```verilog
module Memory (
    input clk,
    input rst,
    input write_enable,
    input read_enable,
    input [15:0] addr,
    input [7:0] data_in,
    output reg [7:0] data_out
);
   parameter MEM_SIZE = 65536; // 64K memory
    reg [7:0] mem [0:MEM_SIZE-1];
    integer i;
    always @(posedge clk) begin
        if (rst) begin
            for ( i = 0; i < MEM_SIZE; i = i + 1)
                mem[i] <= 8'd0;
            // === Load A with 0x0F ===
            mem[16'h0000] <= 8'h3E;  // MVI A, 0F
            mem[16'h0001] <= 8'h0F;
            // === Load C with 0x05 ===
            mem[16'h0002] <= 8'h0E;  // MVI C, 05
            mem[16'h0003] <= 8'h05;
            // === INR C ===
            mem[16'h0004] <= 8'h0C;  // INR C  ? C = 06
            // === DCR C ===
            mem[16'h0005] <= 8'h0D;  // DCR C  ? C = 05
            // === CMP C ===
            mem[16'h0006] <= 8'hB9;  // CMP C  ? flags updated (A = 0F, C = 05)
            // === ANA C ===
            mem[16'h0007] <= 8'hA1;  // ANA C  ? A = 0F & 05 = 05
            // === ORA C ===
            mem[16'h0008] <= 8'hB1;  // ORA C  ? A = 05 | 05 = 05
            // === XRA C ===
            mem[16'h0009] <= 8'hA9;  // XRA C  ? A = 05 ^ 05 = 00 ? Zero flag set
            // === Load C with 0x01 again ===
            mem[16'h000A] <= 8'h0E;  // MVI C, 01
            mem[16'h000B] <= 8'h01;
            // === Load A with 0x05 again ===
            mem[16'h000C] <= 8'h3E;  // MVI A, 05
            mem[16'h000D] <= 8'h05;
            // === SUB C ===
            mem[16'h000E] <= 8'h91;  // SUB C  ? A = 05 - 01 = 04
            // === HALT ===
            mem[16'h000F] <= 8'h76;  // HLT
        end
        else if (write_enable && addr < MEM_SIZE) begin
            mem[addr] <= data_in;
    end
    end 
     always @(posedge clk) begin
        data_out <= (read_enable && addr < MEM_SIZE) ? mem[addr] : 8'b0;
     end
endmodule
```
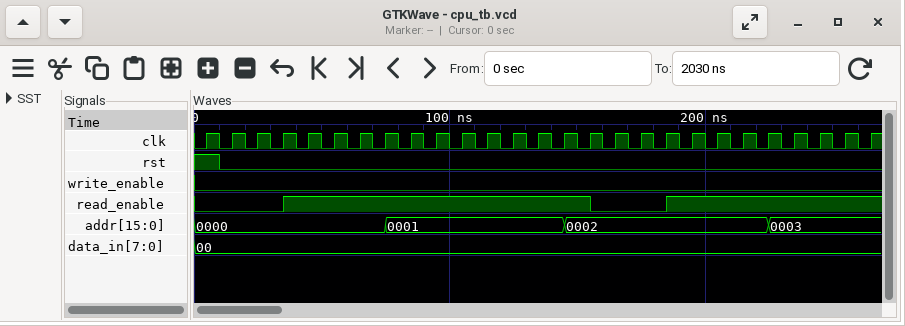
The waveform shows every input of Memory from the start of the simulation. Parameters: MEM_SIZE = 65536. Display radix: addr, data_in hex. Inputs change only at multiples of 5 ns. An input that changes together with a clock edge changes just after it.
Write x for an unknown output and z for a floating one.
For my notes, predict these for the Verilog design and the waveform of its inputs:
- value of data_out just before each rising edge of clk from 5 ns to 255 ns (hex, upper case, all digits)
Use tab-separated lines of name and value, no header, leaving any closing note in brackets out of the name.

value of data_out just before each rising edge of clk from 5 ns to 255 ns	x, 00, 00, 00, 00, 3E, 3E, 3E, 3E, 0F, 0F, 0F, 0F, 0F, 0F, 0F, 0E, 00, 00, 00, 0E, 0E, 0E, 0E, 05, 05
